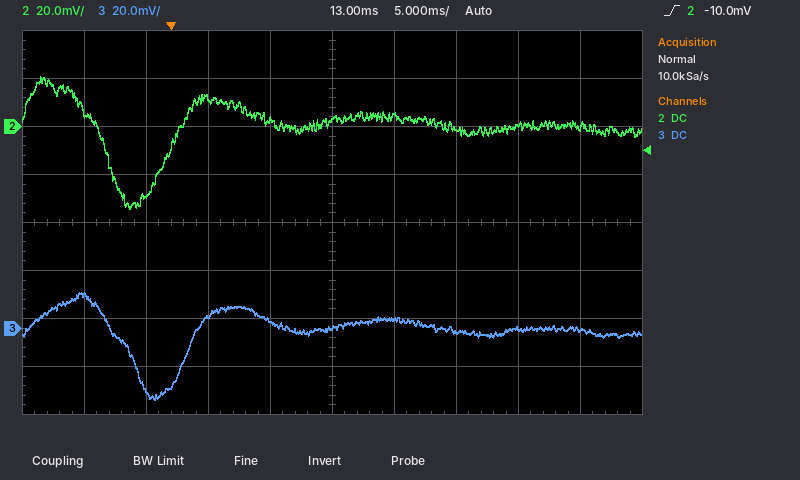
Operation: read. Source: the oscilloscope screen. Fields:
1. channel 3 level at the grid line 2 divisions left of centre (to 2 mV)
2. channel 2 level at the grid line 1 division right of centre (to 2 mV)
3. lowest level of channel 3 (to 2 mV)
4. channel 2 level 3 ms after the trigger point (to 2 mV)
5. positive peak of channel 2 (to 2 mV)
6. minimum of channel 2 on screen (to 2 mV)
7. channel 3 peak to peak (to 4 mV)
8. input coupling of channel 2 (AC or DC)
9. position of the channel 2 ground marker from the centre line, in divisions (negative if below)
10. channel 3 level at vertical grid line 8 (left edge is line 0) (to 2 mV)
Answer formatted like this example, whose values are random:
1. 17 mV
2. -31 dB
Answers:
1. 6 mV
2. 4 mV
3. -30 mV
4. 12 mV
5. 20 mV
6. -34 mV
7. 44 mV
8. DC
9. +2.0 div
10. 0 mV
